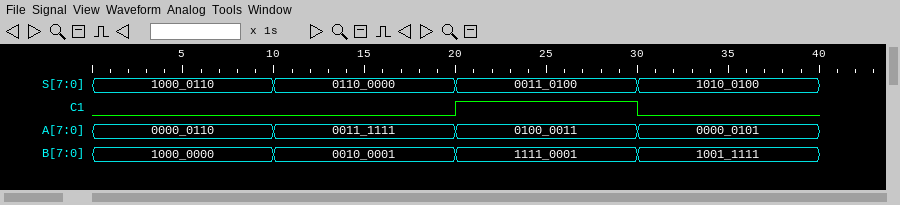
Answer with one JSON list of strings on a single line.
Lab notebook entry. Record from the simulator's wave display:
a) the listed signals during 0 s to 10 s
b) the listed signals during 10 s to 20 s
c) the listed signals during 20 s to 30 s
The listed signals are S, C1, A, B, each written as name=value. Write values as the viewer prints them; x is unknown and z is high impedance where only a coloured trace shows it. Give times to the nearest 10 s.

["S=1000_0110, C1=0, A=0000_0110, B=1000_0000", "S=0110_0000, C1=0, A=0011_1111, B=0010_0001", "S=0011_0100, C1=1, A=0100_0011, B=1111_0001"]
